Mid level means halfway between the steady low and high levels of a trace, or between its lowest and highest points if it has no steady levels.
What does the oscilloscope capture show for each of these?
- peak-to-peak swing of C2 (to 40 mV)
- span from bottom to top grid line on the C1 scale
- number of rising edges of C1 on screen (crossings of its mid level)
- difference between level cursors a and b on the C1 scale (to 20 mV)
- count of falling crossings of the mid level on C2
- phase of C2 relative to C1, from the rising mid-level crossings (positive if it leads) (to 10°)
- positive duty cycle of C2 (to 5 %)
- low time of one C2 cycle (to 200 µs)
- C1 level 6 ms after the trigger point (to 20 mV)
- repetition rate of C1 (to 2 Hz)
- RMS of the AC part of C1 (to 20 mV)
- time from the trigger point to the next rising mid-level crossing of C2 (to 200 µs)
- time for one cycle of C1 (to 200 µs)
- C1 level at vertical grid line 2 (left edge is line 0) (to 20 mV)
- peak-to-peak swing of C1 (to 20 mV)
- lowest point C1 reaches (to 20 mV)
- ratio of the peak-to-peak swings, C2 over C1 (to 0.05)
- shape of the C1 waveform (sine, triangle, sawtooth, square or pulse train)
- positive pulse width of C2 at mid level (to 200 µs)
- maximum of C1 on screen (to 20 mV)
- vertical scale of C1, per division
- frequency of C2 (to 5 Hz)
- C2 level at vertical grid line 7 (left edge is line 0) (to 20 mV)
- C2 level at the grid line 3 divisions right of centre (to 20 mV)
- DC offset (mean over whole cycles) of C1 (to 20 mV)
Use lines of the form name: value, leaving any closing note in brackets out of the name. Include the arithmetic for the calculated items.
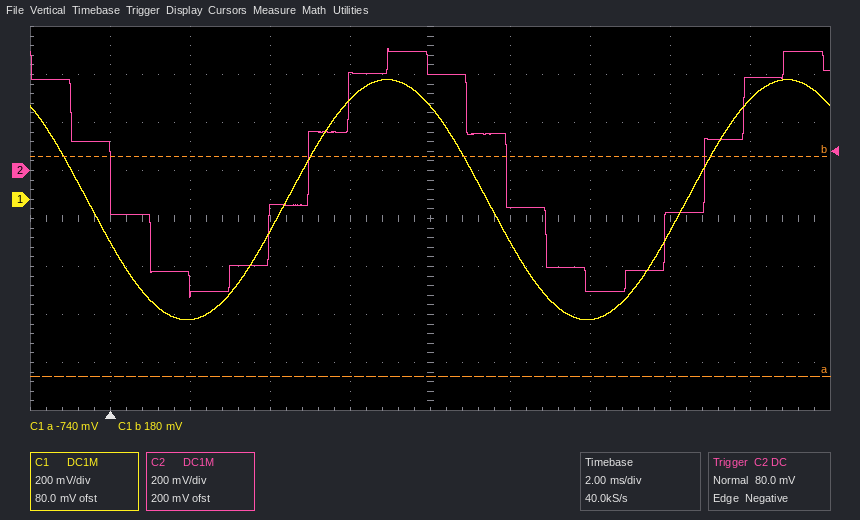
peak-to-peak swing of C2: 1.04 V
span from bottom to top grid line on the C1 scale: 1.6 V
number of rising edges of C1 on screen: 2
difference between level cursors a and b on the C1 scale: 920 mV
count of falling crossings of the mid level on C2: 2
phase of C2 relative to C1, from the rising mid-level crossings (positive if it leads): -20°
positive duty cycle of C2: 50 %
low time of one C2 cycle: 5.0 ms
C1 level 6 ms after the trigger point: 420 mV
repetition rate of C1: 1 / 10.0 ms ≈ 100 Hz
RMS of the AC part of C1: 1.00 V / (2√2) ≈ 354 mV, so 360 mV to the nearest 20 mV
time from the trigger point to the next rising mid-level crossing of C2: 5.0 ms
time for one cycle of C1: 10.0 ms
C1 level at vertical grid line 2 (left edge is line 0): -500 mV
peak-to-peak swing of C1: 500 mV − (-500 mV) = 1.00 V
lowest point C1 reaches: -500 mV
ratio of the peak-to-peak swings, C2 over C1: 1.04 V / 1.00 V ≈ 1.04, so 1.05 to the nearest 0.05
shape of the C1 waveform: sine
positive pulse width of C2 at mid level: 5.0 ms
maximum of C1 on screen: 500 mV
vertical scale of C1, per division: 200 mV
frequency of C2: 100 Hz
C2 level at vertical grid line 7 (left edge is line 0): -500 mV
C2 level at the grid line 3 divisions right of centre: -180 mV
DC offset (mean over whole cycles) of C1: (500 mV + (-500 mV)) / 2 ≈ 0 mV
